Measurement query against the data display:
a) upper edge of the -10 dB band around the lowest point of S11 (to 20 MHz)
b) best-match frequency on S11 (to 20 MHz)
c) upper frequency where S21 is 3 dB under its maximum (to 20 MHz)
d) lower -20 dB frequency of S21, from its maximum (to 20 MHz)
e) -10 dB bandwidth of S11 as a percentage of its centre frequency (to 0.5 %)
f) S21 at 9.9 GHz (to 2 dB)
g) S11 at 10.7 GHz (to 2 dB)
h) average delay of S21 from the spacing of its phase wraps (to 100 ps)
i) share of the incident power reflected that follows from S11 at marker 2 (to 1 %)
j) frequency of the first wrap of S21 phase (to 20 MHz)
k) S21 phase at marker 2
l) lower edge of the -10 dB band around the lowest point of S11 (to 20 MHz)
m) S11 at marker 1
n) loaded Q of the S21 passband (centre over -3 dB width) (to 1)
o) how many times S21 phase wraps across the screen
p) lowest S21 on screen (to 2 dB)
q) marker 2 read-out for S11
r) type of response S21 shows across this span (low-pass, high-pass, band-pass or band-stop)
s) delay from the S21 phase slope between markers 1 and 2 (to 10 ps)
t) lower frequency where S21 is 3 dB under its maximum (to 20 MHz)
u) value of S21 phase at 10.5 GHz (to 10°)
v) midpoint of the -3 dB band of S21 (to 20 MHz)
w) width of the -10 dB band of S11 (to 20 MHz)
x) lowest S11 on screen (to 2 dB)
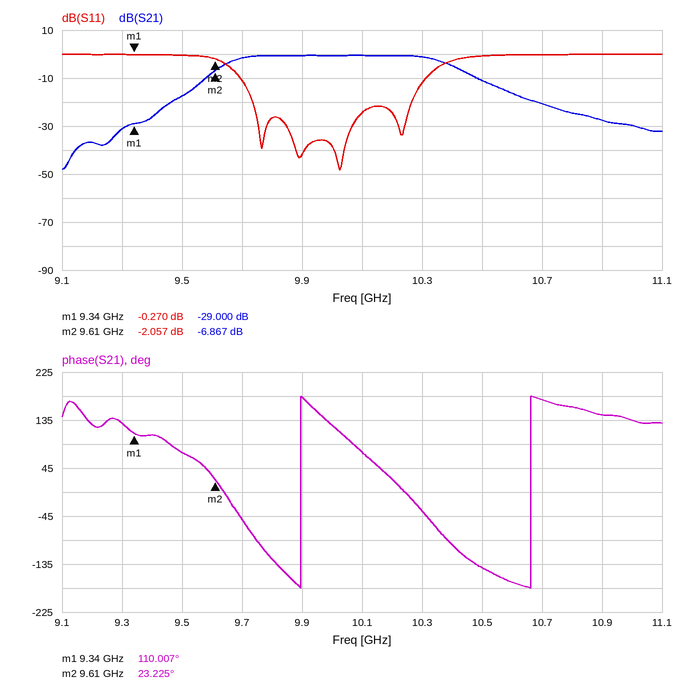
10.32 GHz
10.02 GHz
10.38 GHz
9.46 GHz
6.0 %
0 dB
0 dB
1.3 ns
62 %
9.90 GHz
23.225°
9.70 GHz
-0.270 dB
14
2
-48 dB
-2.057 dB
band-pass
890 ps
9.66 GHz
-140°
10.02 GHz
620 MHz
-48 dB
